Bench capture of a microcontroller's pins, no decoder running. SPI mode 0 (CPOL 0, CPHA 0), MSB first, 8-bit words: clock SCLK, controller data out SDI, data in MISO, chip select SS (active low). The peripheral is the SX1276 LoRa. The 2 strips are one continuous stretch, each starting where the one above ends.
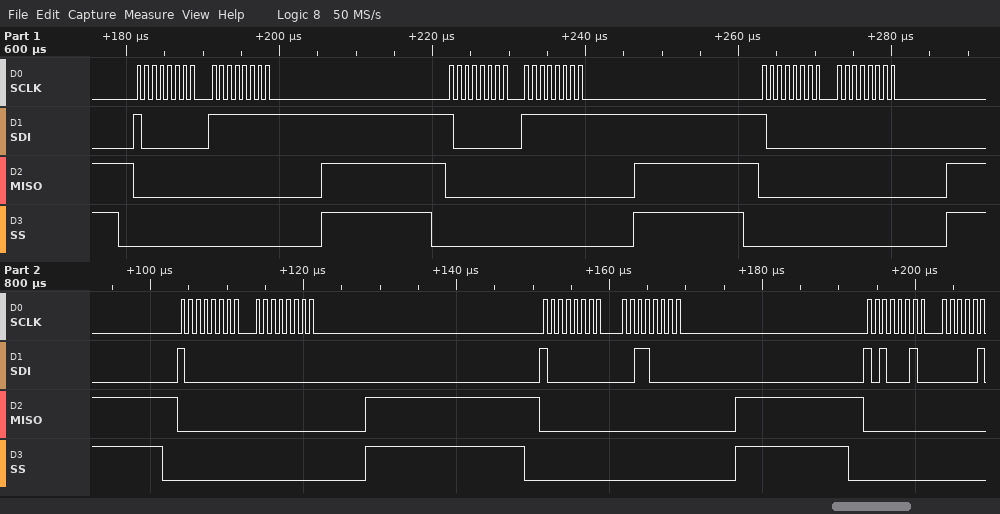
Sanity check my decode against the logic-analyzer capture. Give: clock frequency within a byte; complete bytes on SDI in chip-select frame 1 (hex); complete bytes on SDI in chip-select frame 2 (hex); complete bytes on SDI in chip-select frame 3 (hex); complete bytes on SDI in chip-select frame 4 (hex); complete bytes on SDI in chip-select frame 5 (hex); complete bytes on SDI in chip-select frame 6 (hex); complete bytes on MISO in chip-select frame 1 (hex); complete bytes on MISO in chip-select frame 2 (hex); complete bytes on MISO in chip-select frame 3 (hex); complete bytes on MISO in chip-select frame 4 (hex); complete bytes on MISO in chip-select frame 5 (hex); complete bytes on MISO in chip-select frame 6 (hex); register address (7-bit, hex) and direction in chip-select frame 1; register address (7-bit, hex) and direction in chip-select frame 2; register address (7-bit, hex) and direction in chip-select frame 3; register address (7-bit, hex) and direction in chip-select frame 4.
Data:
1 MHz
80 FF
80 FF
80 00
80 00
80 30
A2
00 00
00 00
00 00
00 00
00 00
00
0x00 write
0x00 write
0x00 write
0x00 write
